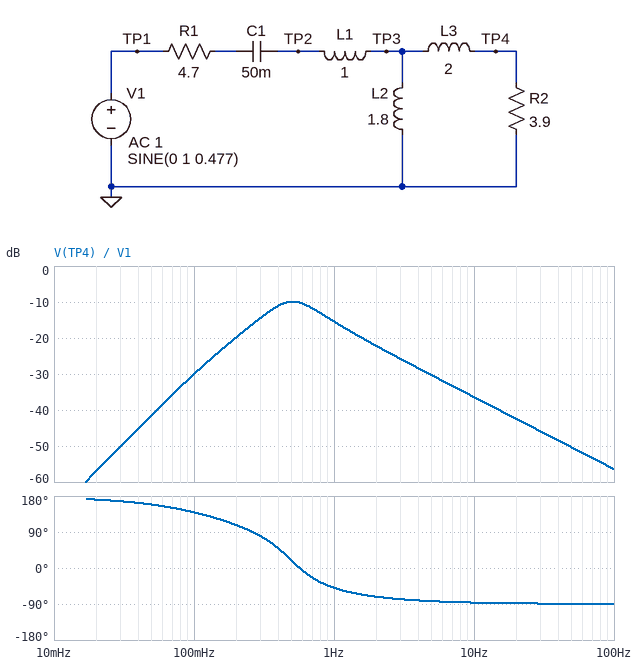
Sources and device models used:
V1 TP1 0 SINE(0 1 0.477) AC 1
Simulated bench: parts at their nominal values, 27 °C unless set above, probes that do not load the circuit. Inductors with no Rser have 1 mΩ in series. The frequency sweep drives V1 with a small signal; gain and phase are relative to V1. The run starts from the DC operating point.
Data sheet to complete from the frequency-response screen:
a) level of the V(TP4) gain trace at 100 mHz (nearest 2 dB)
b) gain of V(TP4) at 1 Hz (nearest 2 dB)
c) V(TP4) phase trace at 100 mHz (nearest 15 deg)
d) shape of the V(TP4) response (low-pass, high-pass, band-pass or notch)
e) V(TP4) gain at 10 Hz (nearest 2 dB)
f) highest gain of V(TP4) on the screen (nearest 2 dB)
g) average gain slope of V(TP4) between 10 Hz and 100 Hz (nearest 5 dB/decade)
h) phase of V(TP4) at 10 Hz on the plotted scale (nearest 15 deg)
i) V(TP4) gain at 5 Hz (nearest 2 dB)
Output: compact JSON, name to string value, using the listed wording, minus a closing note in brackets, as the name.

{"level of the V(TP4) gain trace at 100 mHz": "-30 dB", "gain of V(TP4) at 1 Hz": "-16 dB", "V(TP4) phase trace at 100 mHz": "135 deg", "shape of the V(TP4) response": "band-pass", "V(TP4) gain at 10 Hz": "-36 dB", "highest gain of V(TP4) on the screen": "-10 dB", "average gain slope of V(TP4) between 10 Hz and 100 Hz": "-20 dB/decade", "phase of V(TP4) at 10 Hz on the plotted scale": "-90 deg", "V(TP4) gain at 5 Hz": "-30 dB"}
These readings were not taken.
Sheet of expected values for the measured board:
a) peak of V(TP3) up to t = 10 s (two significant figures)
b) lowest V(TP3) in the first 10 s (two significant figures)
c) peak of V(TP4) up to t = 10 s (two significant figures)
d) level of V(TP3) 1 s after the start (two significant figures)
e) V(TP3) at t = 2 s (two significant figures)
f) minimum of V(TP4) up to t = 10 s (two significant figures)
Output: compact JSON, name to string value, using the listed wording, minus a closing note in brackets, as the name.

{"peak of V(TP3) up to t = 10 s": "580 mV", "lowest V(TP3) in the first 10 s": "-580 mV", "peak of V(TP4) up to t = 10 s": "320 mV", "level of V(TP3) 1 s after the start": "-400 mV", "V(TP3) at t = 2 s": "500 mV", "minimum of V(TP4) up to t = 10 s": "-320 mV"}
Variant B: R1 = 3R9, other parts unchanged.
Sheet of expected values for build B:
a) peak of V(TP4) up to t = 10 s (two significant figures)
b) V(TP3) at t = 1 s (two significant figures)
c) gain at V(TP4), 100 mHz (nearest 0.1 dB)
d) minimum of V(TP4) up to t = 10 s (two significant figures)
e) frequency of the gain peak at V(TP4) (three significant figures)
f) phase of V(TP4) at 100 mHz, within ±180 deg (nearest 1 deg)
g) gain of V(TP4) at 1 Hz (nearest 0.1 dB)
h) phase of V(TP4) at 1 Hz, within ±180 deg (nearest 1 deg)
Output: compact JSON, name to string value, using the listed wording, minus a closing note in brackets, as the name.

{"peak of V(TP4) up to t = 10 s": "370 mV", "V(TP3) at t = 1 s": "-440 mV", "gain at V(TP4), 100 mHz": "-30.0 dB", "minimum of V(TP4) up to t = 10 s": "-370 mV", "frequency of the gain peak at V(TP4)": "504 mHz", "phase of V(TP4) at 100 mHz, within ±180 deg": "141 deg", "gain of V(TP4) at 1 Hz": "-15.1 dB", "phase of V(TP4) at 1 Hz, within ±180 deg": "-53 deg"}
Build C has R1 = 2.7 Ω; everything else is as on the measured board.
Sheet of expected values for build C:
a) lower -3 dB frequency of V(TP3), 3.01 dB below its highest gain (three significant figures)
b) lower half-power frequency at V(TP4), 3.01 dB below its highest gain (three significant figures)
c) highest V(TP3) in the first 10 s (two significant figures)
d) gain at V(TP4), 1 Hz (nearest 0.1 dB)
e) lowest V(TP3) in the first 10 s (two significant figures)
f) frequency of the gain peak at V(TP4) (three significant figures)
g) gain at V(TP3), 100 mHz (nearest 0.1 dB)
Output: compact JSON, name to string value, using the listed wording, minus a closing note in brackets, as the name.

{"lower -3 dB frequency of V(TP3), 3.01 dB below its highest gain": "415 mHz", "lower half-power frequency at V(TP4), 3.01 dB below its highest gain": "383 mHz", "highest V(TP3) in the first 10 s": "910 mV", "gain at V(TP4), 1 Hz": "-14.7 dB", "lowest V(TP3) in the first 10 s": "-910 mV", "frequency of the gain peak at V(TP4)": "502 mHz", "gain at V(TP3), 100 mHz": "-29.5 dB"}
